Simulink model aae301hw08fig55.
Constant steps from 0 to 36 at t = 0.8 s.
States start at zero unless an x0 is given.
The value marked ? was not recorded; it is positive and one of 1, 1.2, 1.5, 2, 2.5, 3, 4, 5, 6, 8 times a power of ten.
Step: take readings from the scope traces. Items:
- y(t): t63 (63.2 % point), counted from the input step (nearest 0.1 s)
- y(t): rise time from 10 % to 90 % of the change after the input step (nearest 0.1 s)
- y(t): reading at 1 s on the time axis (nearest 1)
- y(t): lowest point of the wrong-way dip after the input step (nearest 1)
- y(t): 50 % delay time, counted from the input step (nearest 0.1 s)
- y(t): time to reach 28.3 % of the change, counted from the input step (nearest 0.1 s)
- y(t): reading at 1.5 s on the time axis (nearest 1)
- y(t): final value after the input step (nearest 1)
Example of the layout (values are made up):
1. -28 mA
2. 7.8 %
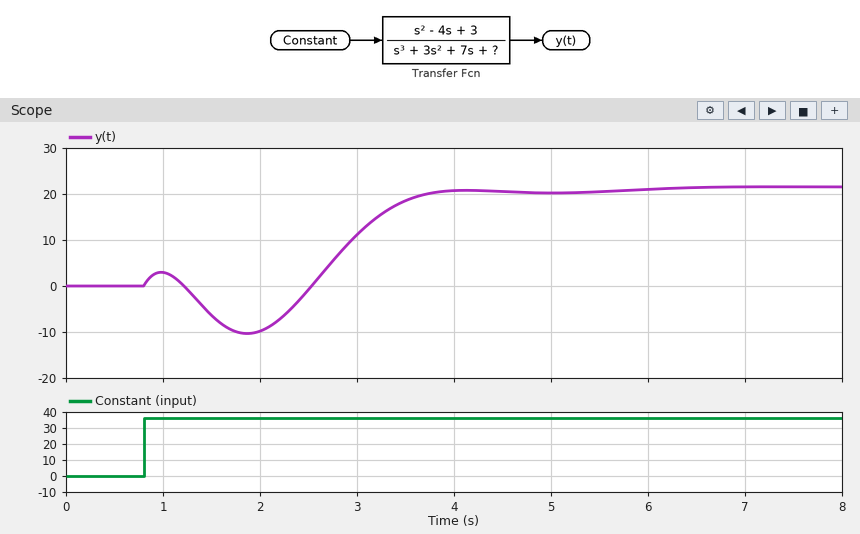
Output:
1. 2.3 s
2. 2.7 s
3. 3
4. -10
5. 2.2 s
6. 2.0 s
7. -6
8. 22
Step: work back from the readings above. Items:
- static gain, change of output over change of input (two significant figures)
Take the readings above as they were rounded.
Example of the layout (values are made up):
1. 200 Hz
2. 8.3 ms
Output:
1. 0.61
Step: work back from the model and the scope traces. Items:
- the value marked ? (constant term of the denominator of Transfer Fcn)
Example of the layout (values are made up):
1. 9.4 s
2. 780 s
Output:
1. 5
